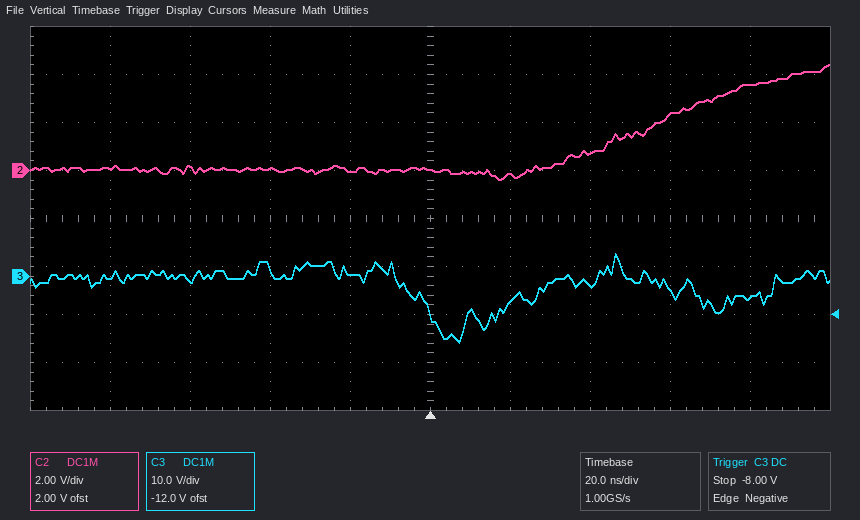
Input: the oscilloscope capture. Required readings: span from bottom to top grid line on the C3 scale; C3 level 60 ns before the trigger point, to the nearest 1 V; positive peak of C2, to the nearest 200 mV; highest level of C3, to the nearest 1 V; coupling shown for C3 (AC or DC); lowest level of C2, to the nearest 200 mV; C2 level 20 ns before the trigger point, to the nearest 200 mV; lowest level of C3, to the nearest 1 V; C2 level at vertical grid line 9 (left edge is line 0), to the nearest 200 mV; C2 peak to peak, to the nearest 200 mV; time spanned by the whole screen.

80 V
-1 V
4.4 V
5 V
DC
-400 mV
0.0 V
-14 V
3.6 V
4.8 V
200 ns
